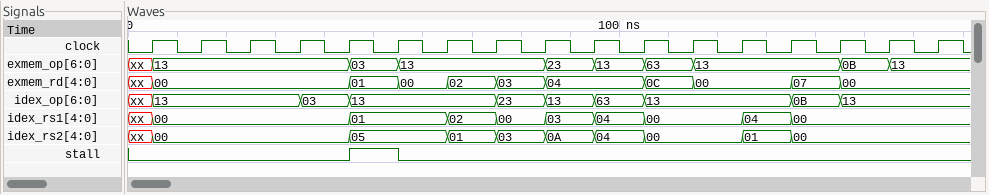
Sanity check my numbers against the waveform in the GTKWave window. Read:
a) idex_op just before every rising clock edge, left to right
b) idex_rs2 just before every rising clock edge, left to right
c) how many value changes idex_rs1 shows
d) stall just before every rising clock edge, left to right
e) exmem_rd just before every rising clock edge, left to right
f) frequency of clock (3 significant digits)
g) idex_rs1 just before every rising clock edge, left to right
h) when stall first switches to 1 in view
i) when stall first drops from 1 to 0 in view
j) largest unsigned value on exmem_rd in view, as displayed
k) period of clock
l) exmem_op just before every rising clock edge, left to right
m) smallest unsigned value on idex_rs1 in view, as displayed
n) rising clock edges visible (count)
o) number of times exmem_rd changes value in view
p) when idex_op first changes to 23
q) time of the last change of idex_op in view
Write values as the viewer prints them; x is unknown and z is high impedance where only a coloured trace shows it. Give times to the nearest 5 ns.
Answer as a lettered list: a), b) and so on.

a) xx, 13, 13, 13, 03, 13, 13, 13, 23, 13, 63, 13, 13, 13, 0B, 13, 13
b) xx, 00, 00, 00, 00, 05, 05, 01, 03, 0A, 04, 00, 00, 01, 00, 00, 00
c) 9
d) 0 0 0 0 0 1 0 0 0 0 0 0 0 0 0 0 0
e) xx, 00, 00, 00, 00, 01, 00, 02, 03, 04, 04, 0C, 00, 00, 07, 00, 00
f) 100 MHz
g) xx, 00, 00, 00, 00, 01, 01, 02, 00, 03, 04, 00, 00, 04, 00, 00, 00
h) 45 ns
i) 55 ns
j) 0C
k) 10 ns
l) xx, 13, 13, 13, 13, 03, 13, 13, 13, 23, 13, 63, 13, 13, 13, 0B, 13
m) 00
n) 17
o) 10
p) 75 ns
q) 145 ns
